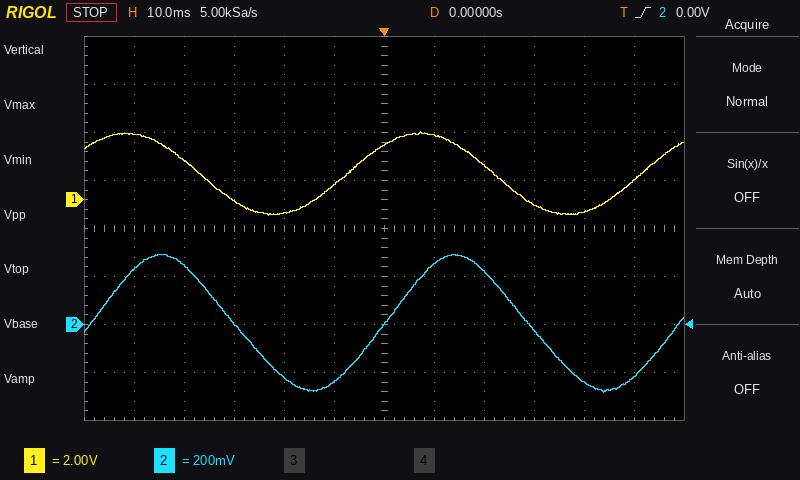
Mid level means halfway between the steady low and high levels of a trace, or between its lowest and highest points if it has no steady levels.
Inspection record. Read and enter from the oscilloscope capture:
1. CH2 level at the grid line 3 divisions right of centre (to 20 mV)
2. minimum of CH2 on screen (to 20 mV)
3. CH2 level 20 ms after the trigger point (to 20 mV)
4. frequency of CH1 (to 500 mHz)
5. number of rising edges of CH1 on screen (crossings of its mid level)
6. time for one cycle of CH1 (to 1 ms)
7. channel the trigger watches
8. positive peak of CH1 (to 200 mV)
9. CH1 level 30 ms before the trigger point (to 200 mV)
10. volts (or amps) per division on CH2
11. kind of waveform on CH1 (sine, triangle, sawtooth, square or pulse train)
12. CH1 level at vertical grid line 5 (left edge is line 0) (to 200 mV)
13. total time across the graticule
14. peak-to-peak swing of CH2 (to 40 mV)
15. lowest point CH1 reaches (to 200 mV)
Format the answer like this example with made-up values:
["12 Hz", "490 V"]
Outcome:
["-20 mV", "-280 mV", "220 mV", "17.0 Hz", "2", "59 ms", "CH2", "2.8 V", "0.0 V", "200 mV", "sine", "600 mV", "120 ms", "560 mV", "-600 mV"]
